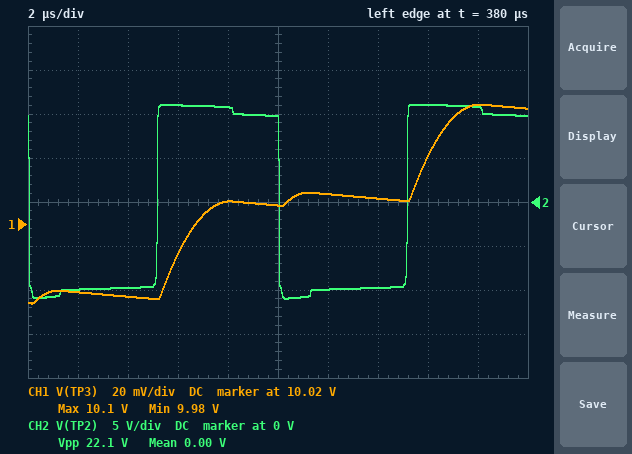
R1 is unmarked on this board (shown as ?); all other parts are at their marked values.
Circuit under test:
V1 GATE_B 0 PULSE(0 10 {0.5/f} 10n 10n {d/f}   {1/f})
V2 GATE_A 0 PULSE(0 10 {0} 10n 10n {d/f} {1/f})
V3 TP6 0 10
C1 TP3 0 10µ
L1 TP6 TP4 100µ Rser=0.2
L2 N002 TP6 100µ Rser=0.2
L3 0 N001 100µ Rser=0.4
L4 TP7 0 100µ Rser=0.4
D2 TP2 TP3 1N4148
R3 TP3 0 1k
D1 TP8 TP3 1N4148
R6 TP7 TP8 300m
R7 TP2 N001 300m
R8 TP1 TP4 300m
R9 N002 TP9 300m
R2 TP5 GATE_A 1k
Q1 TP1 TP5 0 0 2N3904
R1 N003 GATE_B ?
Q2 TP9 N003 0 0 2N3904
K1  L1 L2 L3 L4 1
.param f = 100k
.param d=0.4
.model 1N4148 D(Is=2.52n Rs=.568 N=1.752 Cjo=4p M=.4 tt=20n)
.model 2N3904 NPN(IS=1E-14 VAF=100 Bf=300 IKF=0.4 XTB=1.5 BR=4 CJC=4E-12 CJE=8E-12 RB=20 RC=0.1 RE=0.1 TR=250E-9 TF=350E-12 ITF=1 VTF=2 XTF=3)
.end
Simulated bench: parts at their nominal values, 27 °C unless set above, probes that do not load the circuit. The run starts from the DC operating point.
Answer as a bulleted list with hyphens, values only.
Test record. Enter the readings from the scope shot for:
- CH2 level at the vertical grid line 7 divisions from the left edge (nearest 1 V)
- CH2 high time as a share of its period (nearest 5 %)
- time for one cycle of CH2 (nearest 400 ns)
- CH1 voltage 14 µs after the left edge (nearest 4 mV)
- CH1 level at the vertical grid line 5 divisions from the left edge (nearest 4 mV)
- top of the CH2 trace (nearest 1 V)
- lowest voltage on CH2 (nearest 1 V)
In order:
- -10 V
- 50 %
- 10.0 µs
- 10.032 V
- 10.028 V
- 11 V
- -11 V
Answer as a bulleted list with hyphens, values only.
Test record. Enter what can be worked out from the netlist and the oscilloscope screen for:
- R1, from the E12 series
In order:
- 3.3 kΩ
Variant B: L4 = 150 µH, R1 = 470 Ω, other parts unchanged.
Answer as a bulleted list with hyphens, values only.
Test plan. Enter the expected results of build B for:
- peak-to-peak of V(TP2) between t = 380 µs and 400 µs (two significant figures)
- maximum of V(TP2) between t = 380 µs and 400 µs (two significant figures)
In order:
- 24 V
- 13 V
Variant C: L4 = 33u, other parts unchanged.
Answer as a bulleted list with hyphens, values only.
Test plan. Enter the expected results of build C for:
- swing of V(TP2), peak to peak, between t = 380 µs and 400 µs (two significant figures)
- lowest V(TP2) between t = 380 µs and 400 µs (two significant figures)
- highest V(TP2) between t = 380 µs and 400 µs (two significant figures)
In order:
- 31 V
- -19 V
- 11 V
